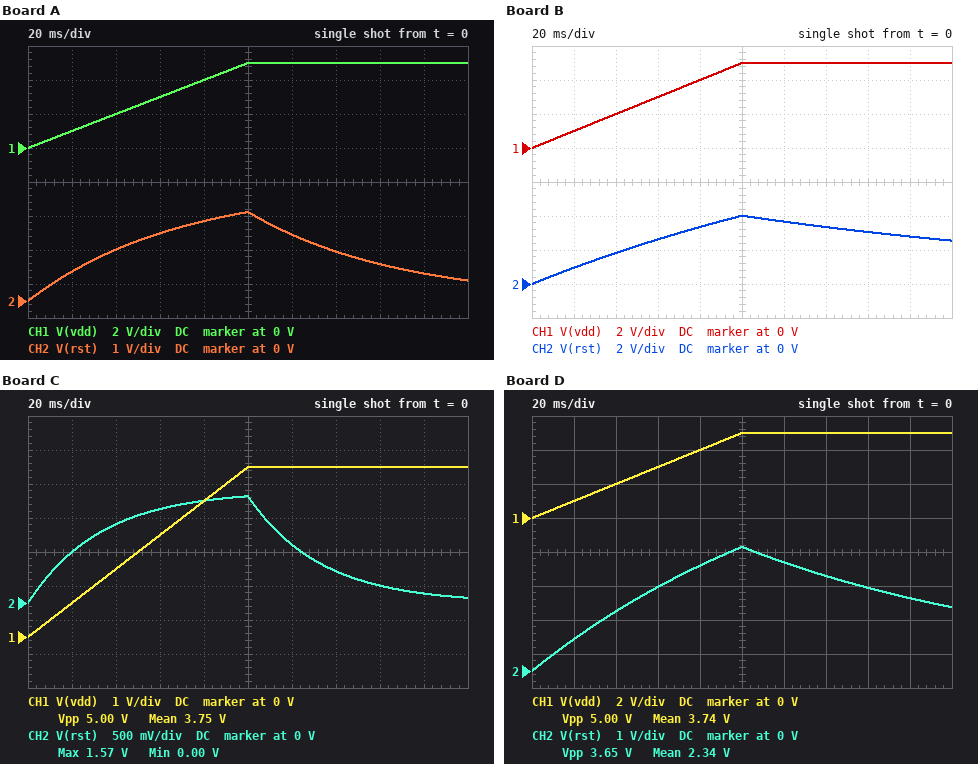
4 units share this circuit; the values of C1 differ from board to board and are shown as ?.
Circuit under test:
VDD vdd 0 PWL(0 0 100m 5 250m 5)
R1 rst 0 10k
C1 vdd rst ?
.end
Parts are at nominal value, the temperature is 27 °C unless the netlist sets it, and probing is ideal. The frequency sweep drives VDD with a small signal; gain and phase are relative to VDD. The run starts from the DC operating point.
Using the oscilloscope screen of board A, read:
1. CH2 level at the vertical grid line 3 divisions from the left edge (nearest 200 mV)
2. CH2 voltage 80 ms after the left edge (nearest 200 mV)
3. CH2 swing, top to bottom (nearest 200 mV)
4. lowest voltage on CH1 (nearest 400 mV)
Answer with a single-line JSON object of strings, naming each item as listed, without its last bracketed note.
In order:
{"CH2 level at the vertical grid line 3 divisions from the left edge": "2.0 V", "CH2 voltage 80 ms after the left edge": "2.4 V", "CH2 swing, top to bottom": "2.6 V", "lowest voltage on CH1": "0 V"}
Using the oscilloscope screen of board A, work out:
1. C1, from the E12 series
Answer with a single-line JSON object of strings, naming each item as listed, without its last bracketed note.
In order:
{"C1, from the E12 series": "6.8 µF"}
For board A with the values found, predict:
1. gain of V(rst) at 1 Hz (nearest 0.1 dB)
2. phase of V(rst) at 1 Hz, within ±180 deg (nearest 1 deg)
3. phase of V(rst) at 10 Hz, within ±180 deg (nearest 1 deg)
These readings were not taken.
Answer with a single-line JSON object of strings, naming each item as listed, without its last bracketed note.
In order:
{"gain of V(rst) at 1 Hz": "-8.1 dB", "phase of V(rst) at 1 Hz, within ±180 deg": "67 deg", "phase of V(rst) at 10 Hz, within ±180 deg": "13 deg"}
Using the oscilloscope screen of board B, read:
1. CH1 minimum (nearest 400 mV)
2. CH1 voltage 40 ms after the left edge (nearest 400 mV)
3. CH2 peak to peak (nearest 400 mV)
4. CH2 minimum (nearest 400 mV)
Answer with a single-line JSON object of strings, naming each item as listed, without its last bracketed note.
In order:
{"CH1 minimum": "0 V", "CH1 voltage 40 ms after the left edge": "2.0 V", "CH2 peak to peak": "4.0 V", "CH2 minimum": "0 V"}
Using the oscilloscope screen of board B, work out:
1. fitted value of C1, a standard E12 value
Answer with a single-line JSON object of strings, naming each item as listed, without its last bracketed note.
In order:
{"fitted value of C1, a standard E12 value": "22 µF"}
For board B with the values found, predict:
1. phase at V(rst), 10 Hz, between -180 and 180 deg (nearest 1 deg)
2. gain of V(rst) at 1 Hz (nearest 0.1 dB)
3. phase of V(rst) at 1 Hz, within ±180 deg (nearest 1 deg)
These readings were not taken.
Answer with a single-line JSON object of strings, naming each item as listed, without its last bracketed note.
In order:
{"phase at V(rst), 10 Hz, between -180 and 180 deg": "4 deg", "gain of V(rst) at 1 Hz": "-1.8 dB", "phase of V(rst) at 1 Hz, within ±180 deg": "36 deg"}
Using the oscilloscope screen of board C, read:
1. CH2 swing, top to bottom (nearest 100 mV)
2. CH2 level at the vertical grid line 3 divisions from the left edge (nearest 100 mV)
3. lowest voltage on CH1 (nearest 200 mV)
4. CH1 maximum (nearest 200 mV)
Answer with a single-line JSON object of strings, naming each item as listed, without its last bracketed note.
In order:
{"CH2 swing, top to bottom": "1.6 V", "CH2 level at the vertical grid line 3 divisions from the left edge": "1.4 V", "lowest voltage on CH1": "0 V", "CH1 maximum": "5.0 V"}
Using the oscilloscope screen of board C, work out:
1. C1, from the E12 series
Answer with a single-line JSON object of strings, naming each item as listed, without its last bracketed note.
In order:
{"C1, from the E12 series": "3.3 µF"}
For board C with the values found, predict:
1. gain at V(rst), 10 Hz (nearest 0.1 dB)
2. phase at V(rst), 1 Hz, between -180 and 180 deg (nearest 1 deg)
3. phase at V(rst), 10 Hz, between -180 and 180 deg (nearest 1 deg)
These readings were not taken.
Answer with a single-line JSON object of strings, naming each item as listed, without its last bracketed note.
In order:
{"gain at V(rst), 10 Hz": "-0.9 dB", "phase at V(rst), 1 Hz, between -180 and 180 deg": "78 deg", "phase at V(rst), 10 Hz, between -180 and 180 deg": "26 deg"}
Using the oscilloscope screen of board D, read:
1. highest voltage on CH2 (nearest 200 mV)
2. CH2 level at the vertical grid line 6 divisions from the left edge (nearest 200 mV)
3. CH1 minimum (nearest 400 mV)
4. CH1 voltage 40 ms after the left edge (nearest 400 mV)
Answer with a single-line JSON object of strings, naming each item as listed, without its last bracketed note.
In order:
{"highest voltage on CH2": "3.6 V", "CH2 level at the vertical grid line 6 divisions from the left edge": "3.2 V", "CH1 minimum": "0 V", "CH1 voltage 40 ms after the left edge": "2.0 V"}
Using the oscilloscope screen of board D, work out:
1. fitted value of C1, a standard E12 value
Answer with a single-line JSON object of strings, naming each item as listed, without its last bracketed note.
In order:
{"fitted value of C1, a standard E12 value": "15 µF"}
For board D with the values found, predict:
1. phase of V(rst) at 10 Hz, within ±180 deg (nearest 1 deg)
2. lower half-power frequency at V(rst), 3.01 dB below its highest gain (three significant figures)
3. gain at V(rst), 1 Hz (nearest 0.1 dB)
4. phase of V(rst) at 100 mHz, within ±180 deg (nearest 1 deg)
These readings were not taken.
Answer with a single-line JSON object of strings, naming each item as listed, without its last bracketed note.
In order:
{"phase of V(rst) at 10 Hz, within ±180 deg": "6 deg", "lower half-power frequency at V(rst), 3.01 dB below its highest gain": "1.06 Hz", "gain at V(rst), 1 Hz": "-3.3 dB", "phase of V(rst) at 100 mHz, within ±180 deg": "85 deg"}
